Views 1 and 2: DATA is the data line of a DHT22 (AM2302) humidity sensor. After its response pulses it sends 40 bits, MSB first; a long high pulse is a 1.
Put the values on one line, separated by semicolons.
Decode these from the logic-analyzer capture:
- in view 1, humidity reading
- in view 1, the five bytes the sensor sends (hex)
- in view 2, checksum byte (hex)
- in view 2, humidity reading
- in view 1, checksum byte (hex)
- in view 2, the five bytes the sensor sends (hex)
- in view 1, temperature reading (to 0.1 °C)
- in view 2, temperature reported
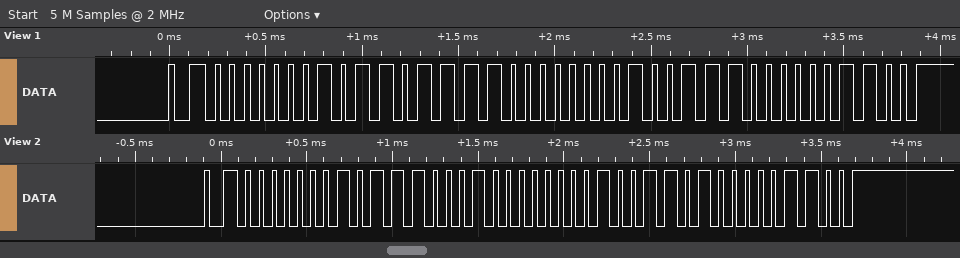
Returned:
36.7 %; 01 6F 00 9C 0C; 0x0C; 36.9 %; 0x0C; 01 71 00 9A 0C; 15.6 °C; 15.4 °C
